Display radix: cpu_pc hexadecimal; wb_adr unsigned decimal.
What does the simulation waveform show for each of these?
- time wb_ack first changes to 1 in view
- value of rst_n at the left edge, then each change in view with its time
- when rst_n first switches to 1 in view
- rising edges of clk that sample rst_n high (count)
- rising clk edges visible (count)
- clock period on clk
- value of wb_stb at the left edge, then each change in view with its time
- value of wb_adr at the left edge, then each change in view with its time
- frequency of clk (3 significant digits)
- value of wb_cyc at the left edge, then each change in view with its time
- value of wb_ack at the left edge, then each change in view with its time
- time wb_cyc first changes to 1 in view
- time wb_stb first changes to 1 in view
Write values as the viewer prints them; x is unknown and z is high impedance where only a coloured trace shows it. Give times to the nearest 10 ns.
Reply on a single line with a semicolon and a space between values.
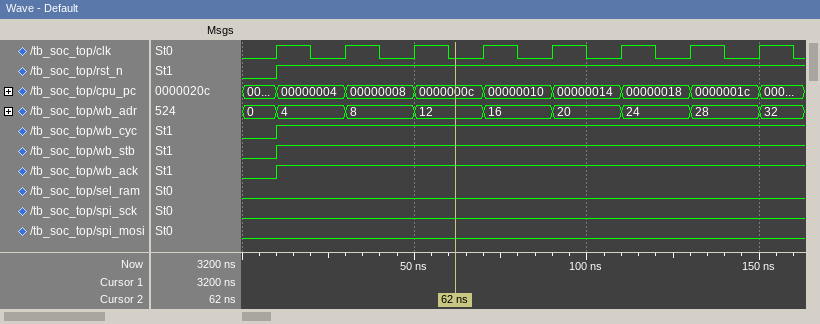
10 ns; 0, 1 at 10 ns; 10 ns; 7; 8; 20 ns; 0, 1 at 10 ns; 0, 4 at 10 ns, 8 at 30 ns, 12 at 50 ns, 16 at 70 ns, 20 at 90 ns, 24 at 110 ns, 28 at 130 ns, 32 at 150 ns; 50.0 MHz; 0, 1 at 10 ns; 0, 1 at 10 ns; 10 ns; 10 ns
